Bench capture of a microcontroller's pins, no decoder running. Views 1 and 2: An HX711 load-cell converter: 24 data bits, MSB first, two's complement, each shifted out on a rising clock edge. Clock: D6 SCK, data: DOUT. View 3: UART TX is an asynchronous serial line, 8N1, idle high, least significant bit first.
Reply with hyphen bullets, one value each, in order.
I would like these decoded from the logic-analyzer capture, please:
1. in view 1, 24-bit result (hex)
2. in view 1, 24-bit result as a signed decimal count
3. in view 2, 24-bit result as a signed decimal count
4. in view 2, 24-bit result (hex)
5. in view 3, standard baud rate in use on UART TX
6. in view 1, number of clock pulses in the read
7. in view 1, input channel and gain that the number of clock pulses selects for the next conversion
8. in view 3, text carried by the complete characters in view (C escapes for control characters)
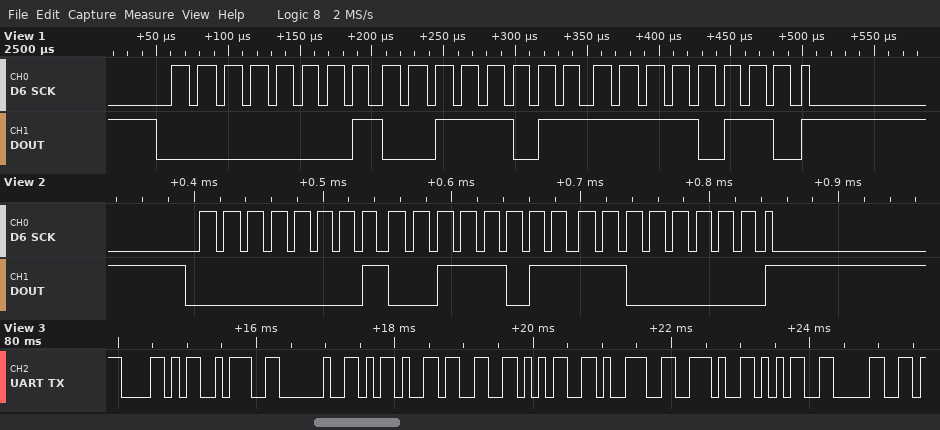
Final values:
- 0x013BF6
- 80886
- 80832
- 0x013BC0
- 9600 baud
- 25
- channel A, gain 128
- "X: -359.50"
